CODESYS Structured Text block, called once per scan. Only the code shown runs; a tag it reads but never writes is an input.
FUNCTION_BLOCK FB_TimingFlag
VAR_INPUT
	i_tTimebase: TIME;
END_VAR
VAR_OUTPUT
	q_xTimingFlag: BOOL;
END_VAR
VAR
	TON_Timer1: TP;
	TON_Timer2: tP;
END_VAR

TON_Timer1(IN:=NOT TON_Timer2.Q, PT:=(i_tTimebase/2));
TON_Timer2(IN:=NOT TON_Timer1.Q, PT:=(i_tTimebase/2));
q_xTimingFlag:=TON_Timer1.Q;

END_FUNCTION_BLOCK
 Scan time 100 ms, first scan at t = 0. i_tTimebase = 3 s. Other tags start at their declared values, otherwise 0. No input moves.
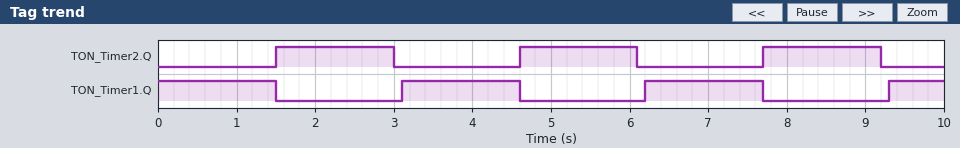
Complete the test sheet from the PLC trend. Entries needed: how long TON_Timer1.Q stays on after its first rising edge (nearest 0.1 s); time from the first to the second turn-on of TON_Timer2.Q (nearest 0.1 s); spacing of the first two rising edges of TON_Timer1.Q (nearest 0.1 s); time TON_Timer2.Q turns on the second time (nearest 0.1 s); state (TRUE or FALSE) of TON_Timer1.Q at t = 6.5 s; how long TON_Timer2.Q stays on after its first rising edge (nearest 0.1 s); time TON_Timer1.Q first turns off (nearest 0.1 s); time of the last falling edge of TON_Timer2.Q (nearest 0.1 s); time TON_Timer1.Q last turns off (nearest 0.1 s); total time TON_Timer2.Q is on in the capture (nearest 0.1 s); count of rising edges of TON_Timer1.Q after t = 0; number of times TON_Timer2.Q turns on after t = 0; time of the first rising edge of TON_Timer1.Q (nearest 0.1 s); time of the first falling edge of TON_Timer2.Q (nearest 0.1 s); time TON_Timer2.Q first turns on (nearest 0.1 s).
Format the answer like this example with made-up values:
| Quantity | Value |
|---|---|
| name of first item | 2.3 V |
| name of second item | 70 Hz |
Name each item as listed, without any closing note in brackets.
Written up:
| Quantity | Value |
|---|---|
| how long TON_Timer1.Q stays on after its first rising edge | 1.5 s |
| time from the first to the second turn-on of TON_Timer2.Q | 3.1 s |
| spacing of the first two rising edges of TON_Timer1.Q | 3.1 s |
| time TON_Timer2.Q turns on the second time | 4.6 s |
| state (TRUE or FALSE) of TON_Timer1.Q at t = 6.5 s | TRUE |
| how long TON_Timer2.Q stays on after its first rising edge | 1.5 s |
| time TON_Timer1.Q first turns off | 1.5 s |
| time of the last falling edge of TON_Timer2.Q | 9.2 s |
| time TON_Timer1.Q last turns off | 7.7 s |
| total time TON_Timer2.Q is on in the capture | 4.5 s |
| count of rising edges of TON_Timer1.Q after t = 0 | 3 |
| number of times TON_Timer2.Q turns on after t = 0 | 3 |
| time of the first rising edge of TON_Timer1.Q | 3.1 s |
| time of the first falling edge of TON_Timer2.Q | 3.0 s |
| time TON_Timer2.Q first turns on | 1.5 s |
